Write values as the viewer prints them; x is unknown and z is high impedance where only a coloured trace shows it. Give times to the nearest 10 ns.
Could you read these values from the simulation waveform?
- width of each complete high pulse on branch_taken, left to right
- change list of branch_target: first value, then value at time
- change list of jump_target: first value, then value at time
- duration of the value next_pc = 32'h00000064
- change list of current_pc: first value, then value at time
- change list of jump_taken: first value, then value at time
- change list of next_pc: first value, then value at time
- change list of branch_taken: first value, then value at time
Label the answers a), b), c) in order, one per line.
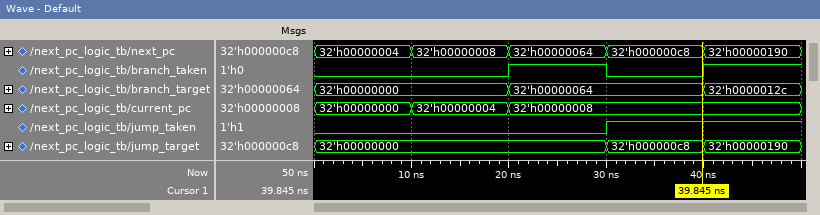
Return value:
a) 10 ns
b) 32'h00000000, 32'h00000064 at 20 ns, 32'h0000012c at 40 ns
c) 32'h00000000, 32'h000000c8 at 30 ns, 32'h00000190 at 40 ns
d) 10 ns
e) 32'h00000000, 32'h00000004 at 10 ns, 32'h00000008 at 20 ns
f) 0, 1 at 30 ns
g) 32'h00000004, 32'h00000008 at 10 ns, 32'h00000064 at 20 ns, 32'h000000c8 at 30 ns, 32'h00000190 at 40 ns
h) 0, 1 at 20 ns, 0 at 30 ns, 1 at 40 ns
